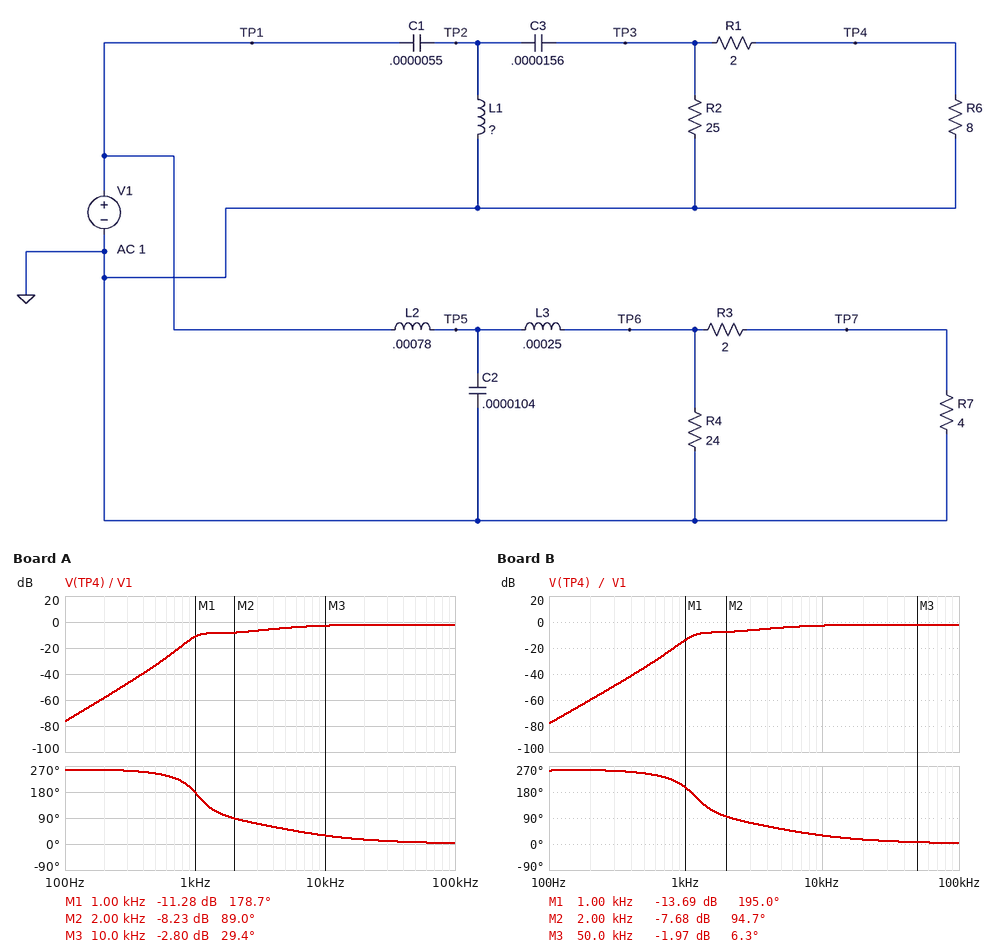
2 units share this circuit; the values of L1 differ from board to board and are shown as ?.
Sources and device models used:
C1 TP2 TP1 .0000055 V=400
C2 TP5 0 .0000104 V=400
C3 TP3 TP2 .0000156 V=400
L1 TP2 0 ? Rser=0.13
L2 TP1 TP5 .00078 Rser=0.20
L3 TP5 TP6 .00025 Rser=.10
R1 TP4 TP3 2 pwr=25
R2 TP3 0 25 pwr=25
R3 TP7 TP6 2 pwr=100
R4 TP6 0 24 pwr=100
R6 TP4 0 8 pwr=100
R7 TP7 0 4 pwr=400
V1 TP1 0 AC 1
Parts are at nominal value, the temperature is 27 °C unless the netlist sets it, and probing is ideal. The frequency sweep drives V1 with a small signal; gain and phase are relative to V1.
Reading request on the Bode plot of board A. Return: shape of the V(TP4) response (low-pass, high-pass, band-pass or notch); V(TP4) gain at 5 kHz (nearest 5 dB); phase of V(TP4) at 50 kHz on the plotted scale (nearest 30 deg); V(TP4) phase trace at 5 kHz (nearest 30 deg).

high-pass
-5 dB
0 deg
60 deg
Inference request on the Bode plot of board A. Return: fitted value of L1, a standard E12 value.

1.2 mH
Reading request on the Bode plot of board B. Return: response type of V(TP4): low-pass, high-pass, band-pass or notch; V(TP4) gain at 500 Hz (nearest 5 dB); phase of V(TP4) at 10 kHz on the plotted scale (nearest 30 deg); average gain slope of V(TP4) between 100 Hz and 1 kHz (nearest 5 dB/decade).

high-pass
-35 dB
30 deg
65 dB/decade
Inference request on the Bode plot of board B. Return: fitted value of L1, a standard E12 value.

1 mH
